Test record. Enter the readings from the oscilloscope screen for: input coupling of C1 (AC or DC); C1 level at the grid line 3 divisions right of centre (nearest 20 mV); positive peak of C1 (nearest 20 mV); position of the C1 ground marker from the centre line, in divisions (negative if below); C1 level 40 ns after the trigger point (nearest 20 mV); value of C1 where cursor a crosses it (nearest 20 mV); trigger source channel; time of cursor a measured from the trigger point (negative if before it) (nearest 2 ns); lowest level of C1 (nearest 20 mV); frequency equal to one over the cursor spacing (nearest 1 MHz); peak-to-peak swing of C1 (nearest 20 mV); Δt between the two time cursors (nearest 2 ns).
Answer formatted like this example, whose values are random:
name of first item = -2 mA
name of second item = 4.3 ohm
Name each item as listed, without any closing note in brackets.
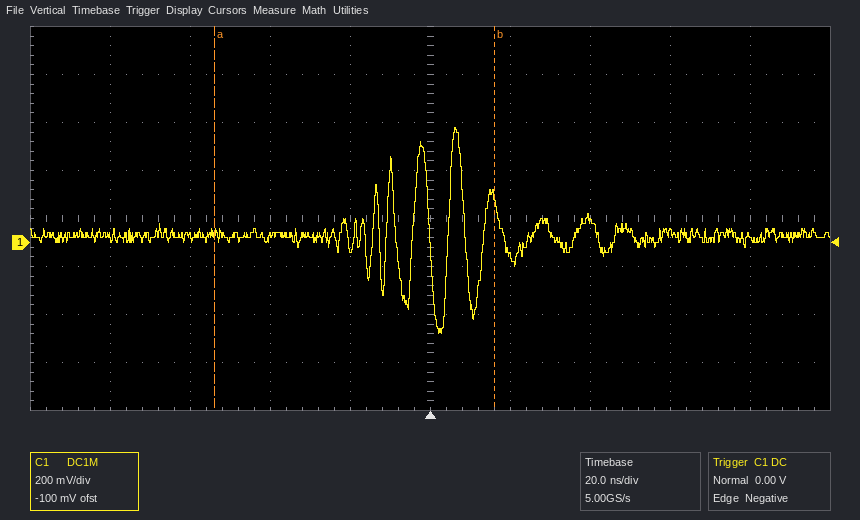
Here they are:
input coupling of C1 = DC
C1 level at the grid line 3 divisions right of centre = 40 mV
positive peak of C1 = 480 mV
position of the C1 ground marker from the centre line, in divisions = -0.5 div
C1 level 40 ns after the trigger point = 100 mV
value of C1 where cursor a crosses it = 40 mV
trigger source channel = C1
time of cursor a measured from the trigger point (negative if before it) = -54 ns
lowest level of C1 = -380 mV
frequency equal to one over the cursor spacing = 14 MHz
peak-to-peak swing of C1 = 860 mV
Δt between the two time cursors = 70 ns
